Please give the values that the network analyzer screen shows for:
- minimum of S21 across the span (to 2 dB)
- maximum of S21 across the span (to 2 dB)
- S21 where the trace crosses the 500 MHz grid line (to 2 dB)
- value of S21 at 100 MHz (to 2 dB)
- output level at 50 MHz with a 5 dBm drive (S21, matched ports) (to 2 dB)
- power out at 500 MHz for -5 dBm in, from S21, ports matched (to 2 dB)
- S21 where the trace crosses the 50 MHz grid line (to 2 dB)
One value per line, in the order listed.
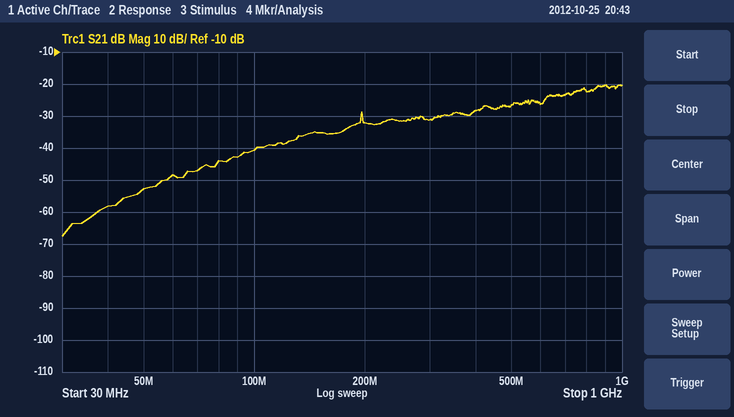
-68 dB
-20 dB
-26 dB
-40 dB
-48 dBm
-32 dBm
-52 dB
